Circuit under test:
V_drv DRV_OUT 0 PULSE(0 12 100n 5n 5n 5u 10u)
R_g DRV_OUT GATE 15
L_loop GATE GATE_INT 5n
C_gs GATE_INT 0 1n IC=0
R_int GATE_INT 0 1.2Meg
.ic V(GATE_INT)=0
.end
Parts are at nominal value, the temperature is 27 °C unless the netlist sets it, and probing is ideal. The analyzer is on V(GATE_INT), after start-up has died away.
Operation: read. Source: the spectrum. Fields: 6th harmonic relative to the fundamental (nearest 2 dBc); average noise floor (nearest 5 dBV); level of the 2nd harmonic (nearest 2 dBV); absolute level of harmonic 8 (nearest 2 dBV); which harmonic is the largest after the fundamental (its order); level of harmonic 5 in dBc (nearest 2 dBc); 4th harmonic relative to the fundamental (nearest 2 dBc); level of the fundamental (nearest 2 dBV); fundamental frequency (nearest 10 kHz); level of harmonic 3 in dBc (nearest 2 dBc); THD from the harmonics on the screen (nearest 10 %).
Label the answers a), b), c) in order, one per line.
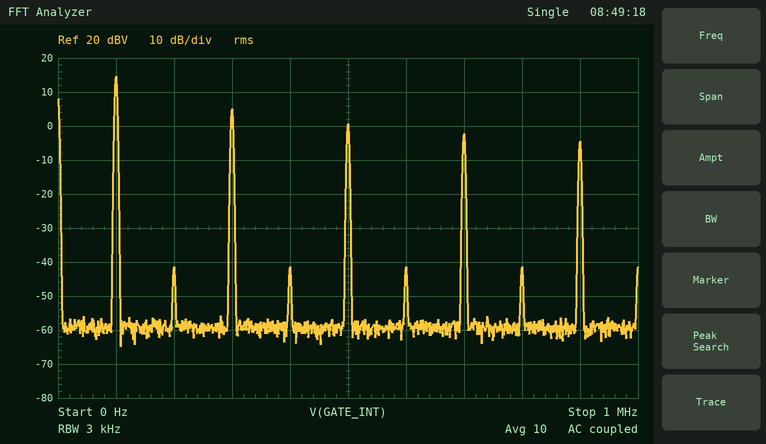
a) -56 dBc
b) -60 dBV
c) -42 dBV
d) -42 dBV
e) 3
f) -14 dBc
g) -56 dBc
h) 14 dBV
i) 100 kHz
j) -10 dBc
k) 40 %
